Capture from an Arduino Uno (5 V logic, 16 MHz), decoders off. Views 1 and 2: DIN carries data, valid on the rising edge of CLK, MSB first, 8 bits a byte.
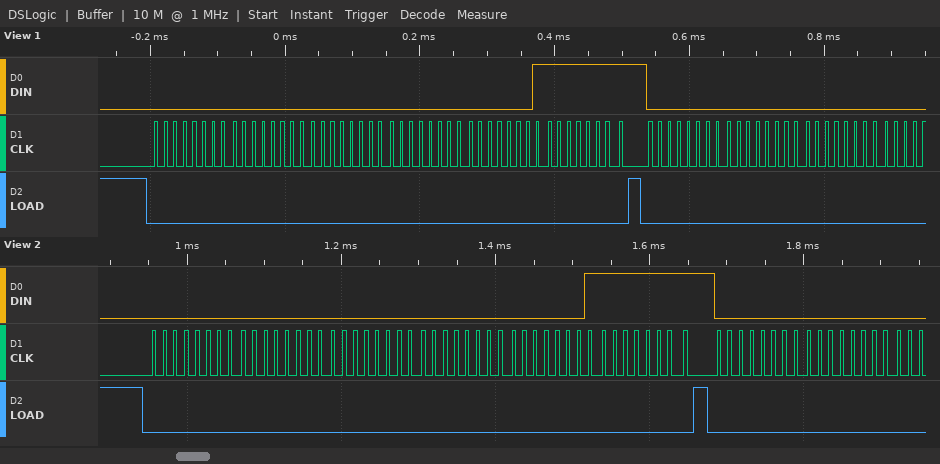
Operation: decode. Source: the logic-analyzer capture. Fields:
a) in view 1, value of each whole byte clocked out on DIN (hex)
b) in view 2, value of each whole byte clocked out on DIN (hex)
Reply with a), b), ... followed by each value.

a) 0x00 0x00 0x00 0x00 0x01 0xFF 0x00 0x00 0x00
b) 00 00 00 00 01 FF 00 00
